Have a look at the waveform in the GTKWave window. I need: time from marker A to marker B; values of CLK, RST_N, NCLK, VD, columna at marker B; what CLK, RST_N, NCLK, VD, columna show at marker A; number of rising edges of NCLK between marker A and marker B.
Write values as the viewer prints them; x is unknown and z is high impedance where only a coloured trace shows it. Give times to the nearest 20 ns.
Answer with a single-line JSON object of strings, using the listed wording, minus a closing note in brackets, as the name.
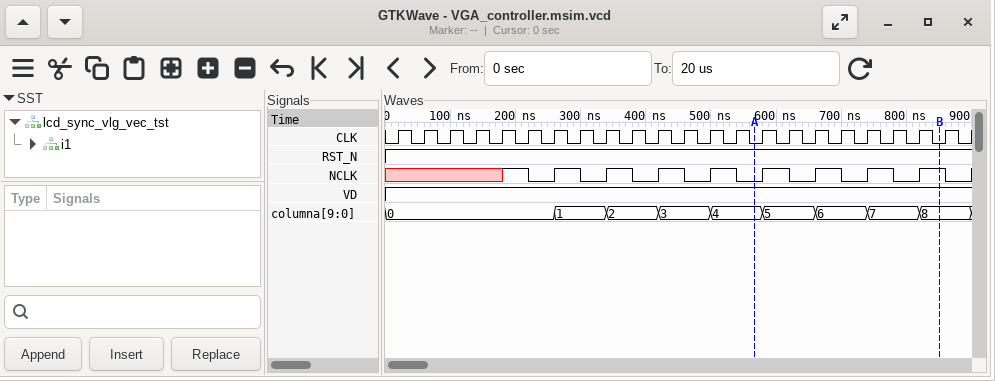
{"time from marker A to marker B": "280 ns", "values of CLK, RST_N, NCLK, VD, columna at marker B": "CLK=0, RST_N=1, NCLK=1, VD=1, columna=8", "what CLK, RST_N, NCLK, VD, columna show at marker A": "CLK=0, RST_N=1, NCLK=0, VD=1, columna=4", "number of rising edges of NCLK between marker A and marker B": "4"}
